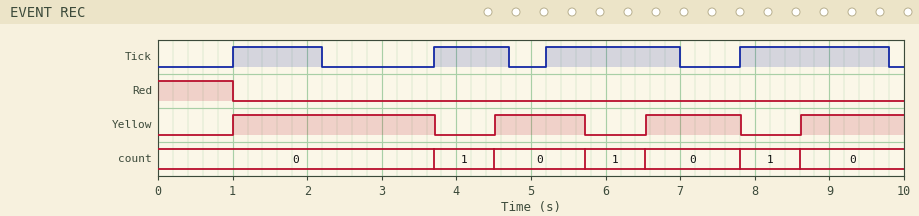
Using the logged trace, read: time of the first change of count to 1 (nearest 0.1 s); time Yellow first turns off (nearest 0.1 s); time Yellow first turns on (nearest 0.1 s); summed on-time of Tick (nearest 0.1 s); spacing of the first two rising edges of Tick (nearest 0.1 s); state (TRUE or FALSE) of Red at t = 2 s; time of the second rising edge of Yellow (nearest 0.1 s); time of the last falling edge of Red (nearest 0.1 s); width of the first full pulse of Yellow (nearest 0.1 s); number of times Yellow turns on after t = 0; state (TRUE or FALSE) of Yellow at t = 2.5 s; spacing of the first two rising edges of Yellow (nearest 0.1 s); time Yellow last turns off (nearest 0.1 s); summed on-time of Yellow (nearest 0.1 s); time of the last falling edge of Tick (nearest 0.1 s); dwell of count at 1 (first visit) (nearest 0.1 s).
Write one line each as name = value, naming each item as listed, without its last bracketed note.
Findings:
time of the first change of count to 1 = 3.7 s
time Yellow first turns off = 3.7 s
time Yellow first turns on = 1.0 s
summed on-time of Tick = 6.0 s
spacing of the first two rising edges of Tick = 2.7 s
state (TRUE or FALSE) of Red at t = 2 s = FALSE
time of the second rising edge of Yellow = 4.5 s
time of the last falling edge of Red = 1.0 s
width of the first full pulse of Yellow = 2.7 s
number of times Yellow turns on after t = 0 = 4
state (TRUE or FALSE) of Yellow at t = 2.5 s = TRUE
spacing of the first two rising edges of Yellow = 3.5 s
time Yellow last turns off = 7.8 s
summed on-time of Yellow = 6.6 s
time of the last falling edge of Tick = 9.8 s
dwell of count at 1 (first visit) = 0.8 s
